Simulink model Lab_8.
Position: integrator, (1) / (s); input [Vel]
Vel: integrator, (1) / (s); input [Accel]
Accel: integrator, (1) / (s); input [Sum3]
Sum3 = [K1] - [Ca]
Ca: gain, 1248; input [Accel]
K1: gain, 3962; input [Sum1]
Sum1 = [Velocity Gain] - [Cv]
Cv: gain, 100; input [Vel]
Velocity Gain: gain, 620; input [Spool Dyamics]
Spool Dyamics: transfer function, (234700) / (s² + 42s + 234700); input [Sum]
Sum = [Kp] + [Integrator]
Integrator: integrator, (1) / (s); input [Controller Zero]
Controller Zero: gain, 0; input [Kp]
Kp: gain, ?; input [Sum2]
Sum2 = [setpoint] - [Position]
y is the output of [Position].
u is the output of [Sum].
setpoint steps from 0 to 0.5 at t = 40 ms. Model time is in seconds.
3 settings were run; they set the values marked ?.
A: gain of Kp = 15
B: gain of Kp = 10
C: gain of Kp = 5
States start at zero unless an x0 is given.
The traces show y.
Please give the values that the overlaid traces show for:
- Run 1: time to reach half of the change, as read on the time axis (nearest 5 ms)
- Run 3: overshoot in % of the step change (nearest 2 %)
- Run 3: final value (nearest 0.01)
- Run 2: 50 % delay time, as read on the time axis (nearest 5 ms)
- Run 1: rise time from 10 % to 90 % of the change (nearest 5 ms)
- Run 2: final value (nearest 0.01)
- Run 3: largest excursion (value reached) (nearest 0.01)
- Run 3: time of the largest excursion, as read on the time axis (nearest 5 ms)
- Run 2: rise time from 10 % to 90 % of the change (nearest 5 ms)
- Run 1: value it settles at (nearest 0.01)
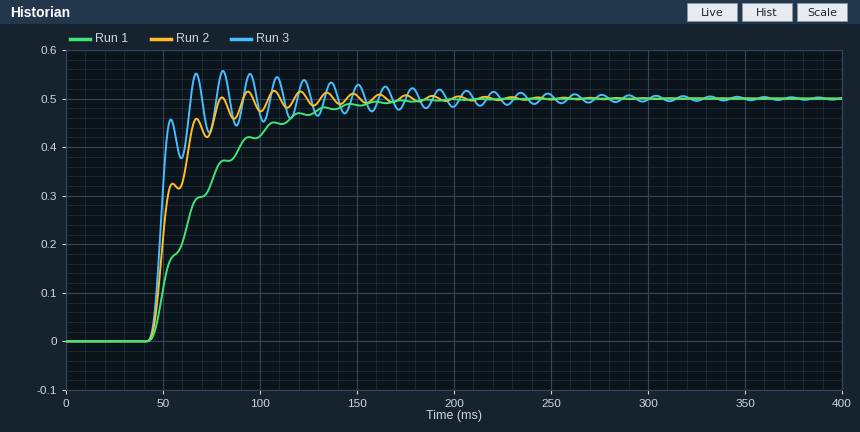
65 ms
12 %
0.50
50 ms
60 ms
0.50
0.56
80 ms
20 ms
0.50
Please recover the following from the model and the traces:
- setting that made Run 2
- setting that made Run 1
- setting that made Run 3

B
C
A
